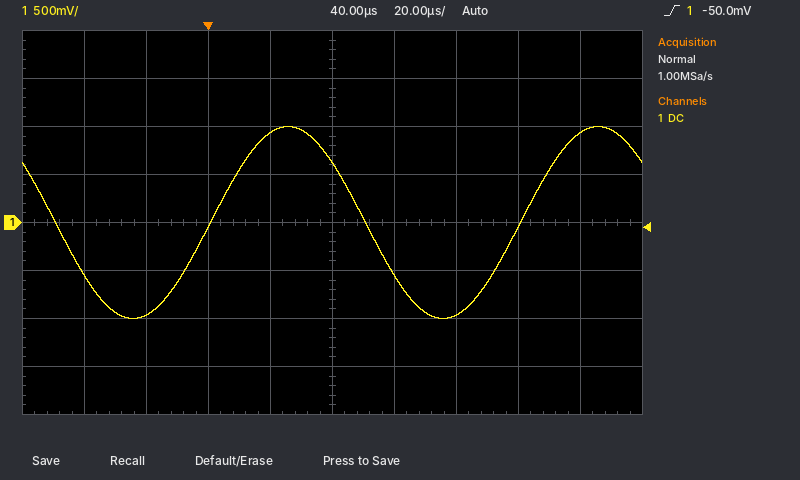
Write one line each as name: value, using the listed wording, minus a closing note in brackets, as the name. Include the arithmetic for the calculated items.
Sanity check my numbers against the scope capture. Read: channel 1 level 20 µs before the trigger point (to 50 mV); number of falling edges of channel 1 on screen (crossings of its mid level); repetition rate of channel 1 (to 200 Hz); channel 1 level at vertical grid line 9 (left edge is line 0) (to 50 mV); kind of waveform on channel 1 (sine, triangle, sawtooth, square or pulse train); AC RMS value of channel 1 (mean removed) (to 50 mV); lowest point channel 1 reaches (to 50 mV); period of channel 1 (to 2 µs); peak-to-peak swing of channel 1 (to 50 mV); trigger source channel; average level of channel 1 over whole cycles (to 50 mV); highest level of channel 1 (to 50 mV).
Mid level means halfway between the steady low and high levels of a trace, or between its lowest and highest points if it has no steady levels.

channel 1 level 20 µs before the trigger point: -950 mV
number of falling edges of channel 1 on screen: 2
repetition rate of channel 1: 1 / 100 µs ≈ 10.0 kHz
channel 1 level at vertical grid line 9 (left edge is line 0): 950 mV
kind of waveform on channel 1: sine
AC RMS value of channel 1 (mean removed): 2.00 V / (2√2) ≈ 707 mV, so 700 mV to the nearest 50 mV
lowest point channel 1 reaches: -1.00 V
period of channel 1: 100 µs
peak-to-peak swing of channel 1: 1.00 V − (-1.00 V) = 2.00 V
trigger source channel: channel 1
average level of channel 1 over whole cycles: (1.00 V + (-1.00 V)) / 2 ≈ 0 mV
highest level of channel 1: 1.00 V
